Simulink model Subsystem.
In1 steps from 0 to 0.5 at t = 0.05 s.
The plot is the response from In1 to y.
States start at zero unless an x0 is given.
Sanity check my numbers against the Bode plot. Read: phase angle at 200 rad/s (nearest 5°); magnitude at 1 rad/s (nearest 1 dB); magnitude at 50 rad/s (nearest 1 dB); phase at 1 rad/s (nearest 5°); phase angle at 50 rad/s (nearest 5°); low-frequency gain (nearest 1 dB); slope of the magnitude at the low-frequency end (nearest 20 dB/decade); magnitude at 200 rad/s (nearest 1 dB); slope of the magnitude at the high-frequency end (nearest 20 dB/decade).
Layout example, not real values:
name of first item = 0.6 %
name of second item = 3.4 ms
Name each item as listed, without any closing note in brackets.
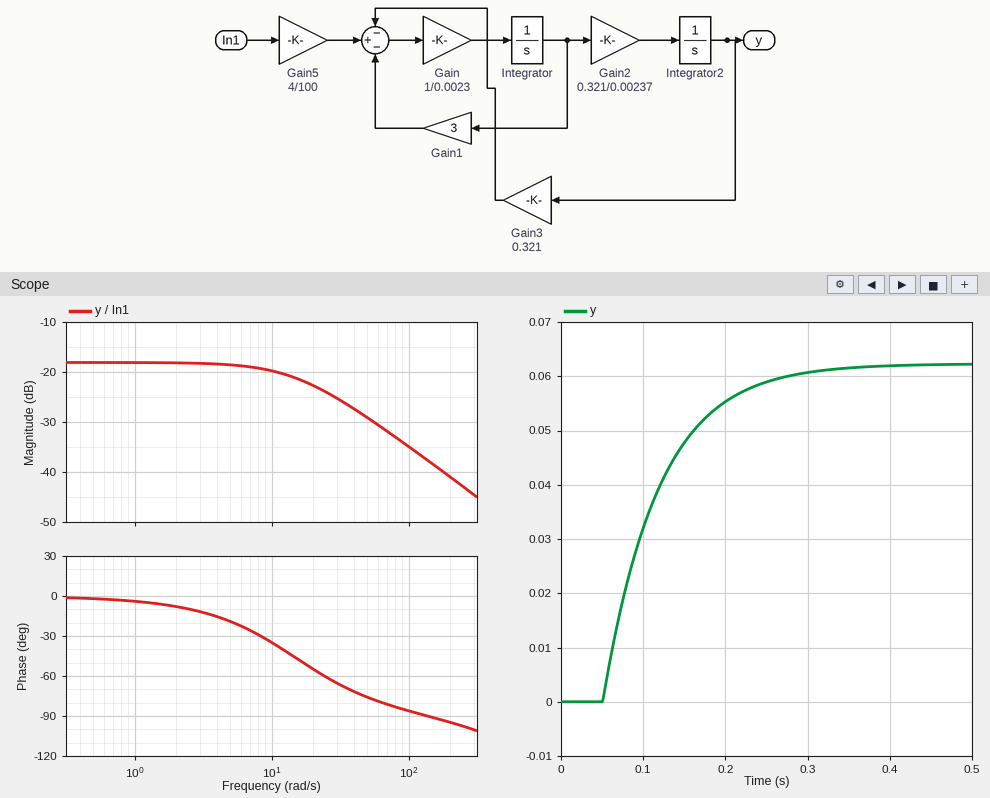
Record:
phase angle at 200 rad/s = -95°
magnitude at 1 rad/s = -18 dB
magnitude at 50 rad/s = -29 dB
phase at 1 rad/s = -5°
phase angle at 50 rad/s = -75°
low-frequency gain = -18 dB
slope of the magnitude at the low-frequency end = 0 dB/decade
magnitude at 200 rad/s = -41 dB
slope of the magnitude at the high-frequency end = -20 dB/decade
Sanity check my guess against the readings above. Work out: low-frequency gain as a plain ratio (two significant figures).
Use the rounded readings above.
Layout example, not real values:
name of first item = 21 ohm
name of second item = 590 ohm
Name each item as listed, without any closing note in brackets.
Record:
low-frequency gain as a plain ratio = 0.13
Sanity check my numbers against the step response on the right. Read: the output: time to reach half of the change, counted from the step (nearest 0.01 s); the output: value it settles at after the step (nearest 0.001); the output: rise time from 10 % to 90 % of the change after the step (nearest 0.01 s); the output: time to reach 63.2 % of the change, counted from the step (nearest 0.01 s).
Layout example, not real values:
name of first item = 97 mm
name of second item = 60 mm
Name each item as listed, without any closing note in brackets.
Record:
the output: time to reach half of the change, counted from the step = 0.05 s
the output: value it settles at after the step = 0.062
the output: rise time from 10 % to 90 % of the change after the step = 0.15 s
the output: time to reach 63.2 % of the change, counted from the step = 0.07 s
